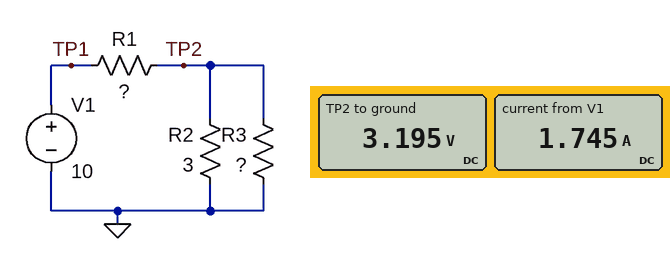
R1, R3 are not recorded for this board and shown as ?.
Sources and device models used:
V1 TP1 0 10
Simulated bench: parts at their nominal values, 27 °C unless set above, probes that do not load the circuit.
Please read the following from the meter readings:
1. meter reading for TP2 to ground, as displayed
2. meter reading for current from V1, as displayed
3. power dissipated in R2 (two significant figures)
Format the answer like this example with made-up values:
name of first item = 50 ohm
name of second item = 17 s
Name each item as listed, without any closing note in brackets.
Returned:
meter reading for TP2 to ground, as displayed = 3.195 V
meter reading for current from V1, as displayed = 1.745 A
power dissipated in R2 = 3.4 W
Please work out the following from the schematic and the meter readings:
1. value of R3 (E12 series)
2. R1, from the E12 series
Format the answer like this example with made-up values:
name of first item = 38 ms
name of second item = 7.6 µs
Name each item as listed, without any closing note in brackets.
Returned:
value of R3 = 4.7 Ω
R1, from the E12 series = 3.9 Ω
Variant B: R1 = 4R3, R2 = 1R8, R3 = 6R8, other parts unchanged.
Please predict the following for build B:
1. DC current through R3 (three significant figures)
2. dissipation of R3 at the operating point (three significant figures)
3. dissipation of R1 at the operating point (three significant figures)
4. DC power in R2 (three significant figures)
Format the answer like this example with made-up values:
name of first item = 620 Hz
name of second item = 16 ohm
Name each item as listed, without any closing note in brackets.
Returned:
DC current through R3 = 366 mA
dissipation of R3 at the operating point = 909 mW
dissipation of R1 at the operating point = 13.1 W
DC power in R2 = 3.44 W
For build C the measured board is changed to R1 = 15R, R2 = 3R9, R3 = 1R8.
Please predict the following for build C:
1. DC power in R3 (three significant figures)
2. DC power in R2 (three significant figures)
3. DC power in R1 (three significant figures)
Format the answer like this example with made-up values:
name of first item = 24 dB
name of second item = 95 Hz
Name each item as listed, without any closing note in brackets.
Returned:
DC power in R3 = 320 mW
DC power in R2 = 148 mW
DC power in R1 = 5.69 W
